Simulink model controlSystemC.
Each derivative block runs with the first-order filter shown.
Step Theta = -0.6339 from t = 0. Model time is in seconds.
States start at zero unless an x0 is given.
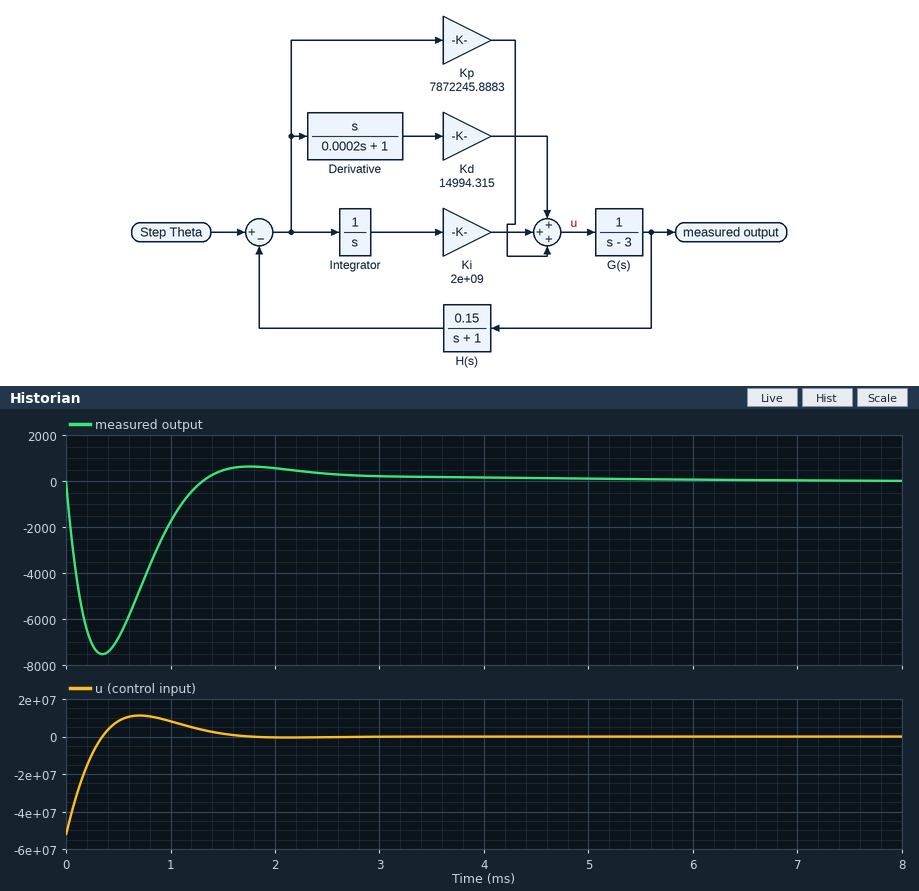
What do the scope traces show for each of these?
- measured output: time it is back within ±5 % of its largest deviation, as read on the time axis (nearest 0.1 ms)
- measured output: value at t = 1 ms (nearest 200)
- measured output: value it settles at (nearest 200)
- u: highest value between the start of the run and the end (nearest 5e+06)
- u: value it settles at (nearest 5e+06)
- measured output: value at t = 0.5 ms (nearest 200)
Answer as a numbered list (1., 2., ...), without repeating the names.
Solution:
1. 2.4 ms
2. -1800
3. 0
4. 10000000
5. 0
6. -6800
